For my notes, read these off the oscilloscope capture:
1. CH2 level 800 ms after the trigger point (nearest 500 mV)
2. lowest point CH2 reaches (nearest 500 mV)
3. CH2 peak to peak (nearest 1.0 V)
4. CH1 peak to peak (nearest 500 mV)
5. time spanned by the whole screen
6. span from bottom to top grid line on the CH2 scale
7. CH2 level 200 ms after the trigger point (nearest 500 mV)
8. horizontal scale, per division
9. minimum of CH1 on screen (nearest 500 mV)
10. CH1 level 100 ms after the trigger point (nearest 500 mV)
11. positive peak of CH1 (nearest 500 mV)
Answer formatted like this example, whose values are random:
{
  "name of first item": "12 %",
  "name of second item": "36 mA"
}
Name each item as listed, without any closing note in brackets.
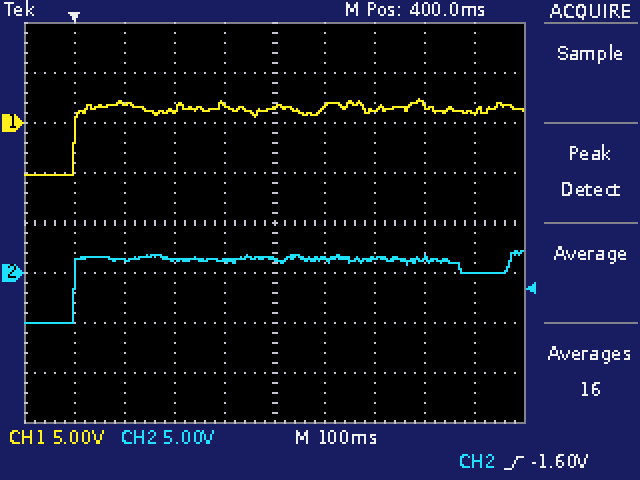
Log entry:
{
  "CH2 level 800 ms after the trigger point": "0.0 V",
  "lowest point CH2 reaches": "-5.0 V",
  "CH2 peak to peak": "7.0 V",
  "CH1 peak to peak": "7.5 V",
  "time spanned by the whole screen": "1 s",
  "span from bottom to top grid line on the CH2 scale": "40 V",
  "CH2 level 200 ms after the trigger point": "1.5 V",
  "horizontal scale, per division": "100 ms",
  "minimum of CH1 on screen": "-5.0 V",
  "CH1 level 100 ms after the trigger point": "2.0 V",
  "positive peak of CH1": "2.5 V"
}
